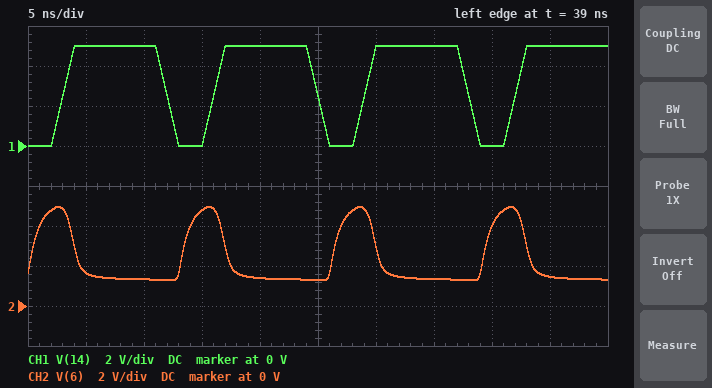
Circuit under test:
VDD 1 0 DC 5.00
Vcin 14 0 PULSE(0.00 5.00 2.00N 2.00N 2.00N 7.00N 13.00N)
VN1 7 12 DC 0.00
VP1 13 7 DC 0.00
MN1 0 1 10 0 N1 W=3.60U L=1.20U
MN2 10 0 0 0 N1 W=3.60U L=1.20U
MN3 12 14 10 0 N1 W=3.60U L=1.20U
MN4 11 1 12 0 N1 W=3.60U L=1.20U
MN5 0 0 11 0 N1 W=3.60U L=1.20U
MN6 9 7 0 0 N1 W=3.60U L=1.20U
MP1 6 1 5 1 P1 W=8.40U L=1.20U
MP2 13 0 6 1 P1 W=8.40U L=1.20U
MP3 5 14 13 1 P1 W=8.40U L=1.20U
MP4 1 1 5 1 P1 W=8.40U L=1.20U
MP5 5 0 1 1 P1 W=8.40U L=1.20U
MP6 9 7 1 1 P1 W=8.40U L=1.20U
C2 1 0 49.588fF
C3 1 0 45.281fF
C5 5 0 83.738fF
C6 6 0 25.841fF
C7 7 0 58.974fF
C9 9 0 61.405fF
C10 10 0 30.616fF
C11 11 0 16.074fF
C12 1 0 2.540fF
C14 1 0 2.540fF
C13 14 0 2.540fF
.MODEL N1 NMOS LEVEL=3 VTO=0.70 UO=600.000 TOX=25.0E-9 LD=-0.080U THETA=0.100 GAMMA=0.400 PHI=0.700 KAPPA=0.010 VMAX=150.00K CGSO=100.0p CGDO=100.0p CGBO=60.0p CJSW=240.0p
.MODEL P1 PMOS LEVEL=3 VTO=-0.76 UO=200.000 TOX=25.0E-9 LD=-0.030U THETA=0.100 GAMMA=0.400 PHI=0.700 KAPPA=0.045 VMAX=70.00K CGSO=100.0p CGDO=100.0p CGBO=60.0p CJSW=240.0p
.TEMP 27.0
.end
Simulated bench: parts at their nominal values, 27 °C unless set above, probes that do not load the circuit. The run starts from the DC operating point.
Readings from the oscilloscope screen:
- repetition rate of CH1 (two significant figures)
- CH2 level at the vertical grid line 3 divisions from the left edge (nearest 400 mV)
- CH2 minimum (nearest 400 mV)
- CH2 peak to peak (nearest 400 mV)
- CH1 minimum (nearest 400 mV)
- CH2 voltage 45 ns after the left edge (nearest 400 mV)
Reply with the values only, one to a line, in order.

77 MHz
4.8 V
1.2 V
3.6 V
0 V
1.6 V
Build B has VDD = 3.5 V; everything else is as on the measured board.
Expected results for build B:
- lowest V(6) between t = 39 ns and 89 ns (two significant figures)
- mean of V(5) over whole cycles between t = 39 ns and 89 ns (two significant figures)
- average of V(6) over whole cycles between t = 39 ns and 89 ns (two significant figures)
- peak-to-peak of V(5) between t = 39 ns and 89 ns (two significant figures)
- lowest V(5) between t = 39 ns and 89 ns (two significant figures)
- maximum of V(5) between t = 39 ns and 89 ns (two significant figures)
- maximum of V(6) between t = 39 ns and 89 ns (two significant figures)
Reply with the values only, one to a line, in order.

1.2 V
3.4 V
1.6 V
670 mV
2.9 V
3.5 V
3.2 V
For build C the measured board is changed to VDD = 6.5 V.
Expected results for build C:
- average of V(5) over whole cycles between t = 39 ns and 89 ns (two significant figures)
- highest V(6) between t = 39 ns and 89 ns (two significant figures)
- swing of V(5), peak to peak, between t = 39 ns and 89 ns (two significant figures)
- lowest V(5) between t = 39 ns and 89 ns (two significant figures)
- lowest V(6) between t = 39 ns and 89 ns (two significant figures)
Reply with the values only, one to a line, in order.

6.3 V
6.5 V
1.1 V
5.4 V
1.4 V
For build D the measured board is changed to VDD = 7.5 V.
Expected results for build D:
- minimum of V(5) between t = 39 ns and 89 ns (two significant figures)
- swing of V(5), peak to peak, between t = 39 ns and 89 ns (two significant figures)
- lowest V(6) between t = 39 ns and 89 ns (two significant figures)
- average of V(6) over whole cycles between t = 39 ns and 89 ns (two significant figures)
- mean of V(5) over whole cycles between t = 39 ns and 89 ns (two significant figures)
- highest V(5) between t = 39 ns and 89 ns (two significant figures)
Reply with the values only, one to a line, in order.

6.3 V
1.2 V
1.5 V
3.7 V
7.2 V
7.5 V
